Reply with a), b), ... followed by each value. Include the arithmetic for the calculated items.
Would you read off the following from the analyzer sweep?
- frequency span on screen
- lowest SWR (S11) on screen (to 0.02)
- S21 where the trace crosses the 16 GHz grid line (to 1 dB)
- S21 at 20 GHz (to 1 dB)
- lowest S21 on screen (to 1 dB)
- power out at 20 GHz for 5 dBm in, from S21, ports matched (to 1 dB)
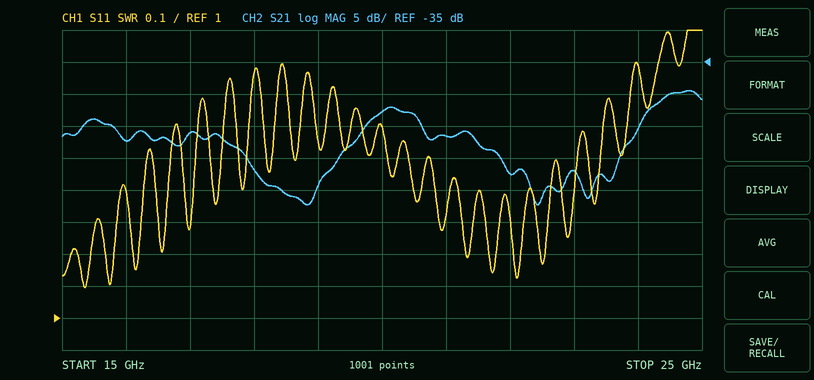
a) 10 GHz
b) 1.10
c) -47 dB
d) -43 dB
e) -57 dB
f) 5 dBm + (-43 dB) = -38 dBm
